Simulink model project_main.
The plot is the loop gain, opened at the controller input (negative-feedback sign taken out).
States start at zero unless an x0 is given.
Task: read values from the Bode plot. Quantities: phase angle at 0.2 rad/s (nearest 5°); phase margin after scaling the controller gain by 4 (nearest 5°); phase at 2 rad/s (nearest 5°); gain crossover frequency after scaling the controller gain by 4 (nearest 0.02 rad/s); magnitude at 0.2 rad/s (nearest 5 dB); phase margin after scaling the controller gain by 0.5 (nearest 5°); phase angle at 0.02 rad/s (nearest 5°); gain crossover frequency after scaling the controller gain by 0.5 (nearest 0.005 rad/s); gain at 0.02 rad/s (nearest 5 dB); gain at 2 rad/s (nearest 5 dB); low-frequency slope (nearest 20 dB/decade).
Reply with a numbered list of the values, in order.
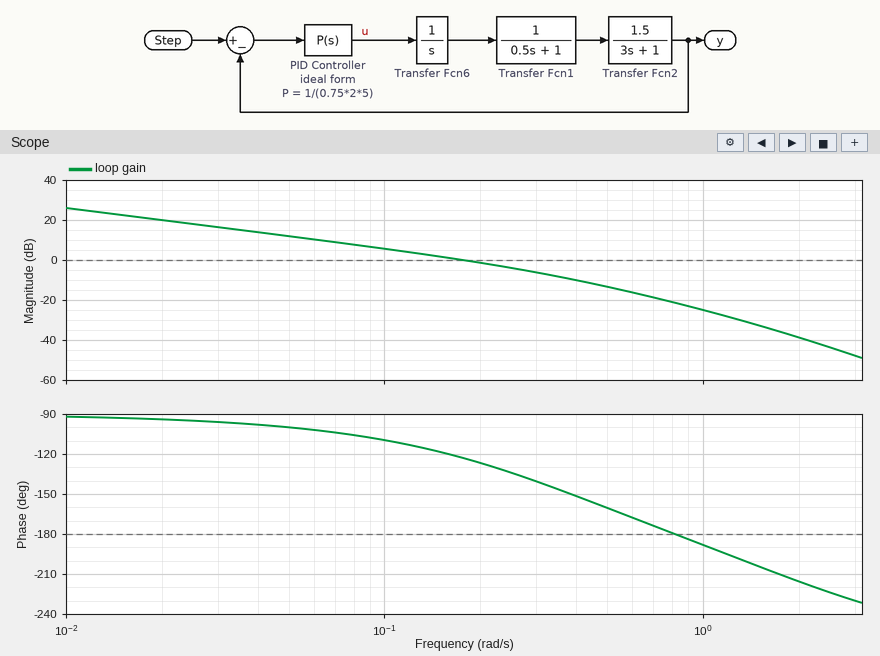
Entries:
1. -125°
2. 25°
3. -215°
4. 0.46 rad/s
5. 0 dB
6. 70°
7. -95°
8. 0.095 rad/s
9. 20 dB
10. -40 dB
11. -20 dB/decade
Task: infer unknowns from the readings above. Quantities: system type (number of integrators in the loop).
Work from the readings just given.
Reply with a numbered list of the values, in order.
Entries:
1. 1
